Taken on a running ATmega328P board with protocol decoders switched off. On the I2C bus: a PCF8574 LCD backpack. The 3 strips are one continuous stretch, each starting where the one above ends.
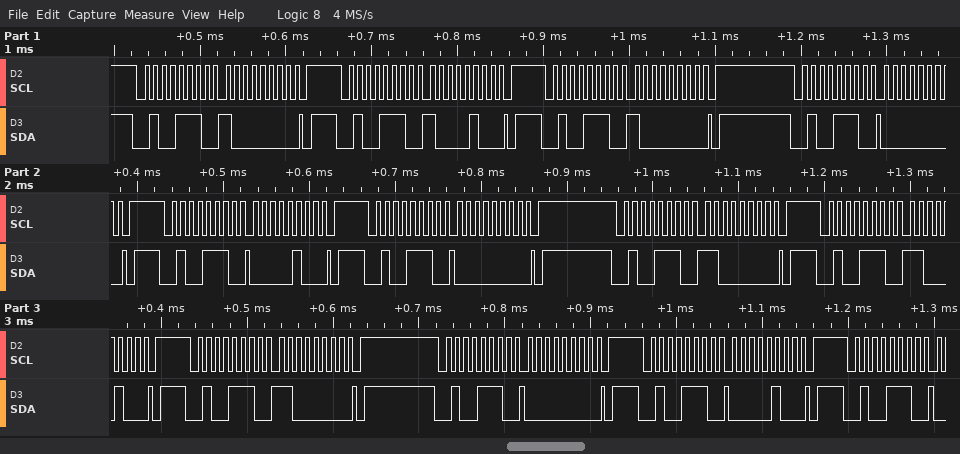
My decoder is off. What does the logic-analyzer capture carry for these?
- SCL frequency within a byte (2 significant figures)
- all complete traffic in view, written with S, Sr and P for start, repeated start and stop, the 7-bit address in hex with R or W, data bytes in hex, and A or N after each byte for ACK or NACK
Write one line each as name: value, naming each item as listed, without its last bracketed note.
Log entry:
SCL frequency within a byte: 100 kHz
all complete traffic in view, written with S, Sr and P for start, repeated start and stop, the 7-bit address in hex with R or W, data bytes in hex, and A or N after each byte for ACK or NACK: S 27W A 80 A P S 27W A 84 A P S 27W A 80 A P S 27W A 00 A P S 27W A 04 A P S 27W A 00 A P S 27W A C0 A P S 27W A C4 A P S 27W A C0 A P S 27W A 00 A P S 27W A 04 A P S 27W A
